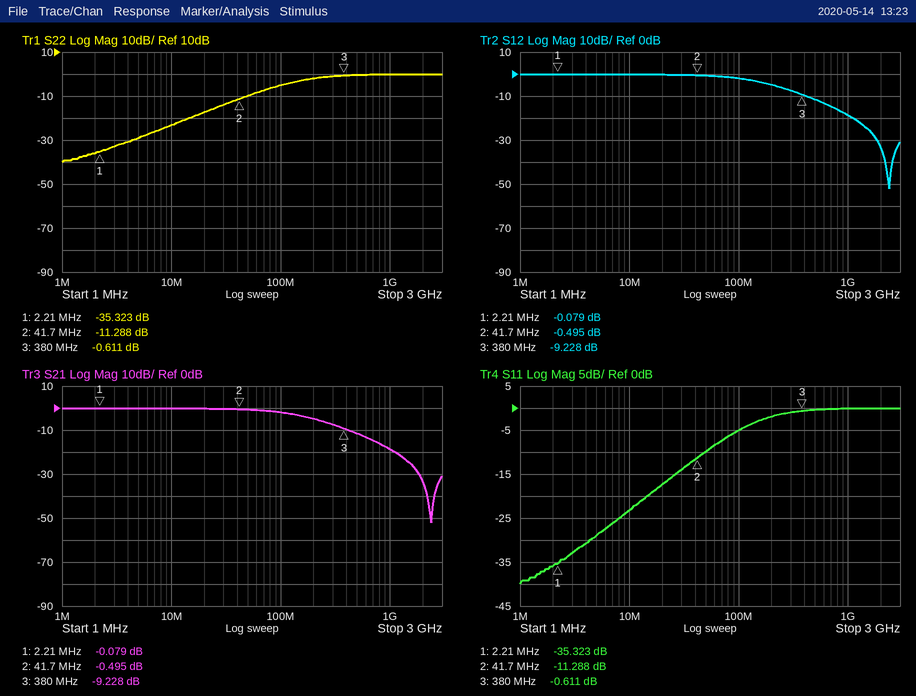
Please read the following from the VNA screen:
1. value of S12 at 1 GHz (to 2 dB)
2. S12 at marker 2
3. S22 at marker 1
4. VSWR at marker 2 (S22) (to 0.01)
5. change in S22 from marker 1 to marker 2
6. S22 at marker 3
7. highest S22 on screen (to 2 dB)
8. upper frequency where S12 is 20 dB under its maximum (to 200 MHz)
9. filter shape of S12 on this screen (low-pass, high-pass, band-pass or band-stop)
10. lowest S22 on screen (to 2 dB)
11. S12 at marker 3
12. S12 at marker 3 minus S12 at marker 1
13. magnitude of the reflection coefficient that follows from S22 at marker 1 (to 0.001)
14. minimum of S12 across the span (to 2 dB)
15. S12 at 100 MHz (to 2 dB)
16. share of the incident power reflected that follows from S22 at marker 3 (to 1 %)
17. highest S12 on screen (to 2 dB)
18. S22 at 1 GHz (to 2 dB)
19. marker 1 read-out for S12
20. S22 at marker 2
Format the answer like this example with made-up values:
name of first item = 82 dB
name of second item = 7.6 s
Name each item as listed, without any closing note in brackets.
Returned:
value of S12 at 1 GHz = -18 dB
S12 at marker 2 = -0.495 dB
S22 at marker 1 = -35.323 dB
VSWR at marker 2 (S22) = 1.75
change in S22 from marker 1 to marker 2 = 24.035 dB
S22 at marker 3 = -0.611 dB
highest S22 on screen = 0 dB
upper frequency where S12 is 20 dB under its maximum = 1.2 GHz
filter shape of S12 on this screen = low-pass
lowest S22 on screen = -40 dB
S12 at marker 3 = -9.228 dB
S12 at marker 3 minus S12 at marker 1 = -9.149 dB
magnitude of the reflection coefficient that follows from S22 at marker 1 = 0.017
minimum of S12 across the span = -52 dB
S12 at 100 MHz = -2 dB
share of the incident power reflected that follows from S22 at marker 3 = 87 %
highest S12 on screen = 0 dB
S22 at 1 GHz = 0 dB
marker 1 read-out for S12 = -0.079 dB
S22 at marker 2 = -11.288 dB
